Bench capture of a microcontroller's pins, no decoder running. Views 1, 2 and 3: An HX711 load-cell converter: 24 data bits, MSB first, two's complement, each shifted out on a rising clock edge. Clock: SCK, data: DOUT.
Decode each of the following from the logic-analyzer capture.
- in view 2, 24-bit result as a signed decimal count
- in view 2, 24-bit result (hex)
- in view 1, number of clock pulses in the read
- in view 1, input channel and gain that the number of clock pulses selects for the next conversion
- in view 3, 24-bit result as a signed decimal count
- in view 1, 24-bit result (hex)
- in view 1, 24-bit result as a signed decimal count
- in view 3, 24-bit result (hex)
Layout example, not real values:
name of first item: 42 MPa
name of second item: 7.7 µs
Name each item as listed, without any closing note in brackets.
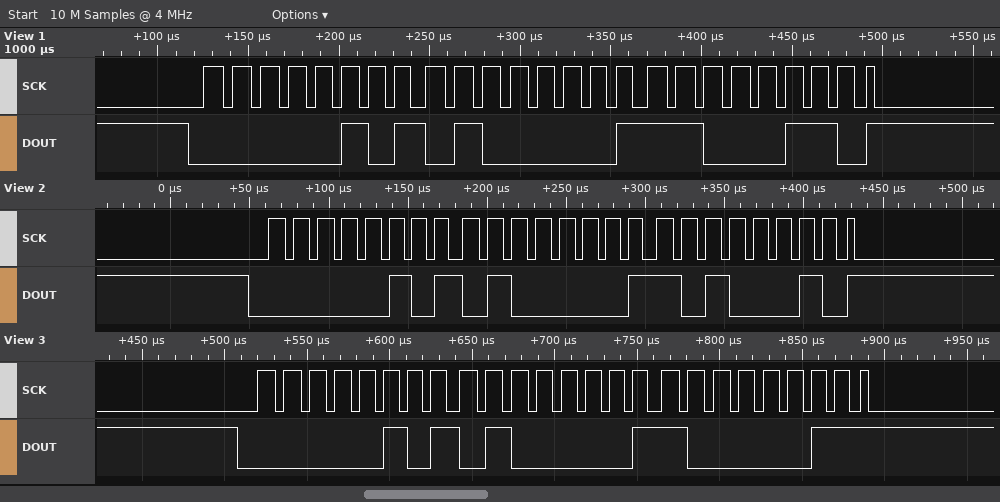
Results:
in view 2, 24-bit result as a signed decimal count: 344482
in view 2, 24-bit result: 0x0541A2
in view 1, number of clock pulses in the read: 25
in view 1, input channel and gain that the number of clock pulses selects for the next conversion: channel A, gain 128
in view 3, 24-bit result as a signed decimal count: 344451
in view 1, 24-bit result: 0x0541C6
in view 1, 24-bit result as a signed decimal count: 344518
in view 3, 24-bit result: 0x054183
